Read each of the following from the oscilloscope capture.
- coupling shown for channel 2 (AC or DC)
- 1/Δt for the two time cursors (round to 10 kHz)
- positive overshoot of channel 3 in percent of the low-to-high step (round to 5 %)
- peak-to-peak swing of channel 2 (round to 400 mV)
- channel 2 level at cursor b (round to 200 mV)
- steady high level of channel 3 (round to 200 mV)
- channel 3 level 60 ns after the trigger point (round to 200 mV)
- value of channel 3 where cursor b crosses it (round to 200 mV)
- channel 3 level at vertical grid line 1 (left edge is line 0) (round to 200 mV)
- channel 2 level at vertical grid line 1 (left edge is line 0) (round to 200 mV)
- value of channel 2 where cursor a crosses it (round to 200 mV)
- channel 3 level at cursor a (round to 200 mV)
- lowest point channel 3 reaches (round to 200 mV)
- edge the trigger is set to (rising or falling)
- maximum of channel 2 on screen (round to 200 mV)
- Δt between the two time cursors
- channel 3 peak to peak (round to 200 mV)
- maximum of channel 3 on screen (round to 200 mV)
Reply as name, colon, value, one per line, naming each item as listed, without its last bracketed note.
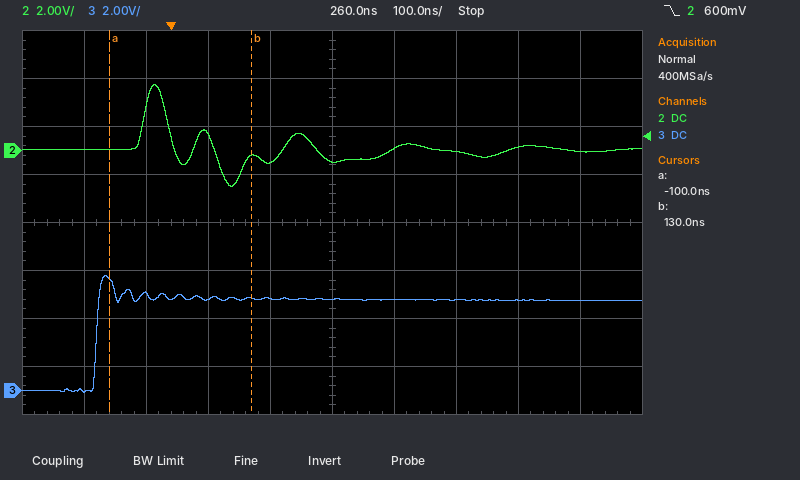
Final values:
coupling shown for channel 2: DC
1/Δt for the two time cursors: 4.35 MHz
positive overshoot of channel 3 in percent of the low-to-high step: 25 %
peak-to-peak swing of channel 2: 4.4 V
channel 2 level at cursor b: -200 mV
steady high level of channel 3: 3.8 V
channel 3 level 60 ns after the trigger point: 3.8 V
value of channel 3 where cursor b crosses it: 3.8 V
channel 3 level at vertical grid line 1 (left edge is line 0): 0.0 V
channel 2 level at vertical grid line 1 (left edge is line 0): 0.0 V
value of channel 2 where cursor a crosses it: 0.0 V
channel 3 level at cursor a: 4.6 V
lowest point channel 3 reaches: 0.0 V
edge the trigger is set to: falling
maximum of channel 2 on screen: 2.8 V
Δt between the two time cursors: 230 ns
channel 3 peak to peak: 4.8 V
maximum of channel 3 on screen: 4.8 V
